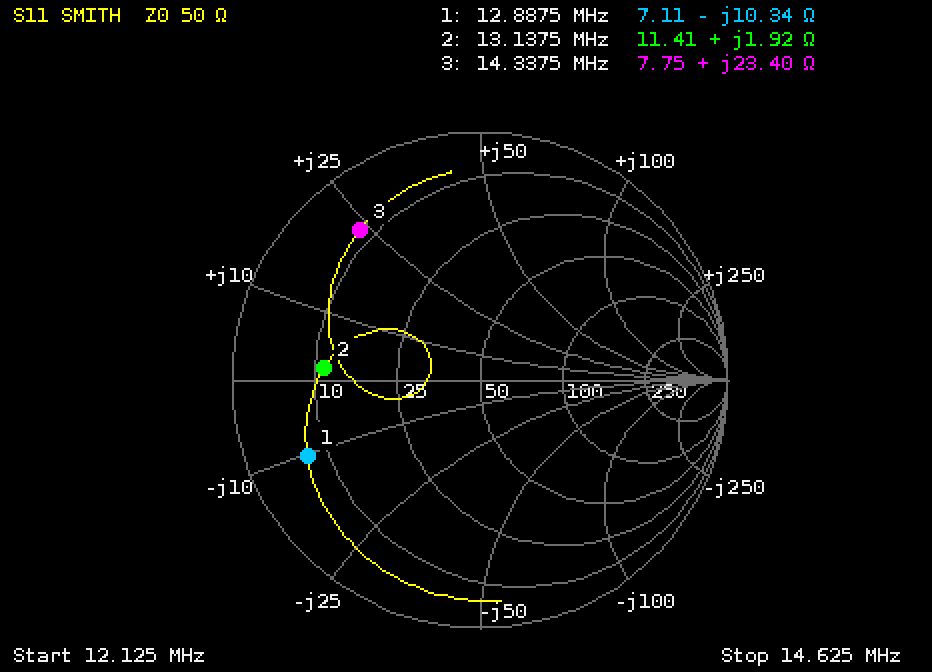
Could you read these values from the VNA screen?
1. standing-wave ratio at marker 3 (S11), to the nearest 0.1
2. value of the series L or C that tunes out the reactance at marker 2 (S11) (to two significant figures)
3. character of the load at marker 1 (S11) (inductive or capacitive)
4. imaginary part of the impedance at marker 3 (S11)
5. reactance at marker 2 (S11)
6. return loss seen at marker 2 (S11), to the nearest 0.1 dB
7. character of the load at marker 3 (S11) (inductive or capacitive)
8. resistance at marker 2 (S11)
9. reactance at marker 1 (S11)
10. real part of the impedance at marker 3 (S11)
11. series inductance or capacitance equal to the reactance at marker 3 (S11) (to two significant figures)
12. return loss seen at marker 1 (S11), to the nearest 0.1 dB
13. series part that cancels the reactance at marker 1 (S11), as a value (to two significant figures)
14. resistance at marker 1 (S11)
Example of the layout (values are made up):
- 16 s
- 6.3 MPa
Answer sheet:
- 7.9
- 6.3 nF
- capacitive
- +23.40 Ω
- +1.92 Ω
- 4.0 dB
- inductive
- 11.41 Ω
- -10.34 Ω
- 7.75 Ω
- 260 nH
- 2.4 dB
- 130 nH
- 7.11 Ω
